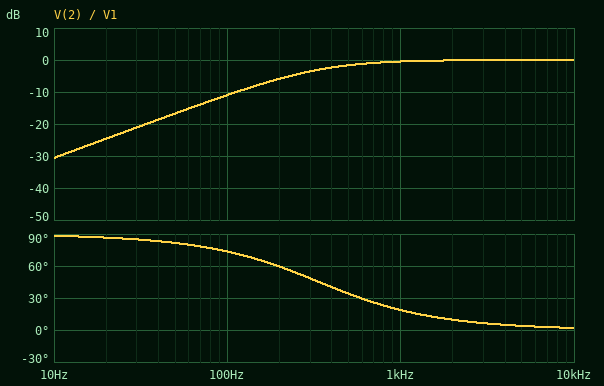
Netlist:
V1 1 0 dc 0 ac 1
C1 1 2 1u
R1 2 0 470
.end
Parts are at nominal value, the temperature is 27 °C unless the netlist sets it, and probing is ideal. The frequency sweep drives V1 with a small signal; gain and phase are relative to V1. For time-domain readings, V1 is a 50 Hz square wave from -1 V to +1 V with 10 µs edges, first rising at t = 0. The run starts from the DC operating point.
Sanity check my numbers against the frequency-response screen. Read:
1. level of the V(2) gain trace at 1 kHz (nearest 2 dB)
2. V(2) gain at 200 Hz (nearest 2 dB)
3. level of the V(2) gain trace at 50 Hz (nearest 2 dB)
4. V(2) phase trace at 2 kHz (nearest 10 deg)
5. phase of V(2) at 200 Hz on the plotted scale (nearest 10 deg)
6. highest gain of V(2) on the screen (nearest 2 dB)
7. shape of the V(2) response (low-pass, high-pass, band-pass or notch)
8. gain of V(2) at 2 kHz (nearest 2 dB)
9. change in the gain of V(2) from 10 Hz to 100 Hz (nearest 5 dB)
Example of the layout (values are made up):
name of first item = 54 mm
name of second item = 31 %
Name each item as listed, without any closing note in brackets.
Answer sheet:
level of the V(2) gain trace at 1 kHz = 0 dB
V(2) gain at 200 Hz = -6 dB
level of the V(2) gain trace at 50 Hz = -16 dB
V(2) phase trace at 2 kHz = 10 deg
phase of V(2) at 200 Hz on the plotted scale = 60 deg
highest gain of V(2) on the screen = 0 dB
shape of the V(2) response = high-pass
gain of V(2) at 2 kHz = 0 dB
change in the gain of V(2) from 10 Hz to 100 Hz = 20 dB
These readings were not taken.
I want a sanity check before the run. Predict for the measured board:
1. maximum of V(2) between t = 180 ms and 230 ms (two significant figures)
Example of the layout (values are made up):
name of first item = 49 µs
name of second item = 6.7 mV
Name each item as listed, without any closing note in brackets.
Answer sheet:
maximum of V(2) between t = 180 ms and 230 ms = 2.0 V
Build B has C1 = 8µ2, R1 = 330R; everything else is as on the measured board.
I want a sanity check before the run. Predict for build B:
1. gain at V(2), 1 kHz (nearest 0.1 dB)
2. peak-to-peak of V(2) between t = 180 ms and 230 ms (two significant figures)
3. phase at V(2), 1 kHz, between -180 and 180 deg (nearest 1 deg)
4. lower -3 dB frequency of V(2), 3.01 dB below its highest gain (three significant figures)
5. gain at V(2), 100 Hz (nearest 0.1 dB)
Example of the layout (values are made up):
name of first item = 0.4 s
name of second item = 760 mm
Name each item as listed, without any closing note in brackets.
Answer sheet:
gain at V(2), 1 kHz = 0 dB
peak-to-peak of V(2) between t = 180 ms and 230 ms = 3.9 V
phase at V(2), 1 kHz, between -180 and 180 deg = 3 deg
lower -3 dB frequency of V(2), 3.01 dB below its highest gain = 58.8 Hz
gain at V(2), 100 Hz = -1.3 dB
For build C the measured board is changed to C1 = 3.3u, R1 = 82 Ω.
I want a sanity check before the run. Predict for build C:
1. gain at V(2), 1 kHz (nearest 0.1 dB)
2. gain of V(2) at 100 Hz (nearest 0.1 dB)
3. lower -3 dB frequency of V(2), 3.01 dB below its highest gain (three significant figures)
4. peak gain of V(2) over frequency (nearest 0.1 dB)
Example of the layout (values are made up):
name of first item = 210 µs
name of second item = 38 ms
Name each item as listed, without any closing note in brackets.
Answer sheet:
gain at V(2), 1 kHz = -1.3 dB
gain of V(2) at 100 Hz = -15.5 dB
lower -3 dB frequency of V(2), 3.01 dB below its highest gain = 588 Hz
peak gain of V(2) over frequency = 0 dB
